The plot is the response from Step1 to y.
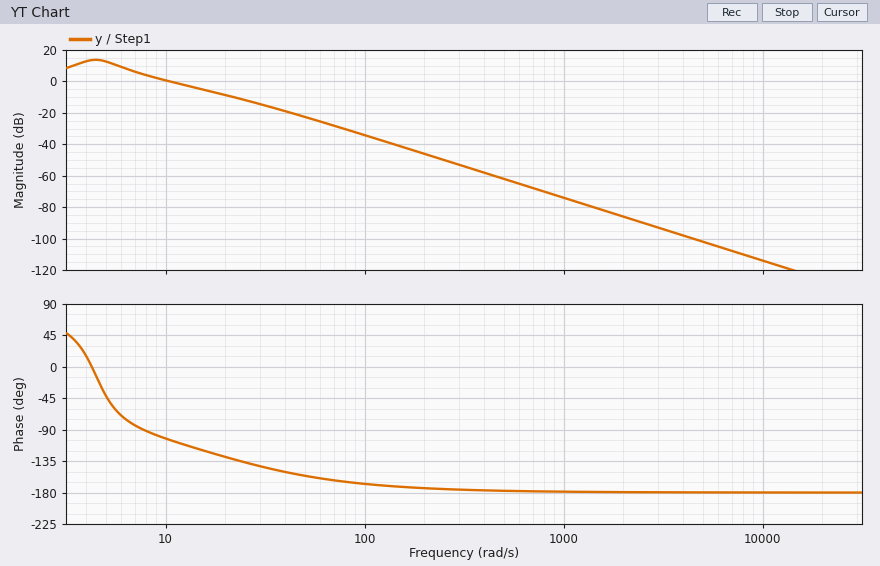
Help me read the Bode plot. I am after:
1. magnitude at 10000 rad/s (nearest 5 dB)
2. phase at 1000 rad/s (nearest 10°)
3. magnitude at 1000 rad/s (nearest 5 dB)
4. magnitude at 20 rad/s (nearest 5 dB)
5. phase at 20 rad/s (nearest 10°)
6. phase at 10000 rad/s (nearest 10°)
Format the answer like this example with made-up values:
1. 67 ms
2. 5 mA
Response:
1. -115 dB
2. -180°
3. -75 dB
4. -10 dB
5. -130°
6. -180°
